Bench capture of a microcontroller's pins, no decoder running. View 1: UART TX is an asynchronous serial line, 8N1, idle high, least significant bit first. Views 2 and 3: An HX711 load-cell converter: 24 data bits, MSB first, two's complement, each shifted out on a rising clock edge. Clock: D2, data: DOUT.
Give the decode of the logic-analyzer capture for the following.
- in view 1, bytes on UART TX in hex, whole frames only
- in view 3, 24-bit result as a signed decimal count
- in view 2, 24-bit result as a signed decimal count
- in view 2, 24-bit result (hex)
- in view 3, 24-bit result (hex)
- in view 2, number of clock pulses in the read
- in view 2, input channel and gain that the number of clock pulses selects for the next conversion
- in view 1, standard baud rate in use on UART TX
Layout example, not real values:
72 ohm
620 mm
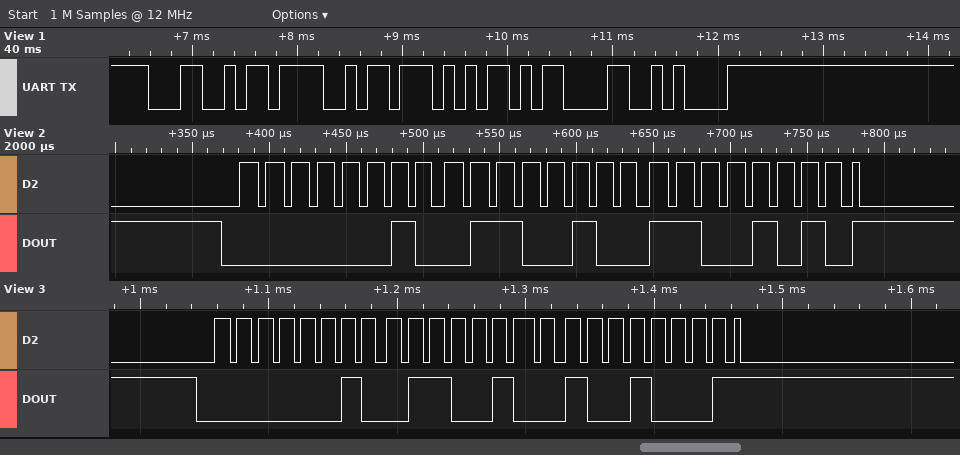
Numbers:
4C 4F 57 0D 0A
156817
156874
0x0264CA
0x026491
25
channel A, gain 128
9600 baud
